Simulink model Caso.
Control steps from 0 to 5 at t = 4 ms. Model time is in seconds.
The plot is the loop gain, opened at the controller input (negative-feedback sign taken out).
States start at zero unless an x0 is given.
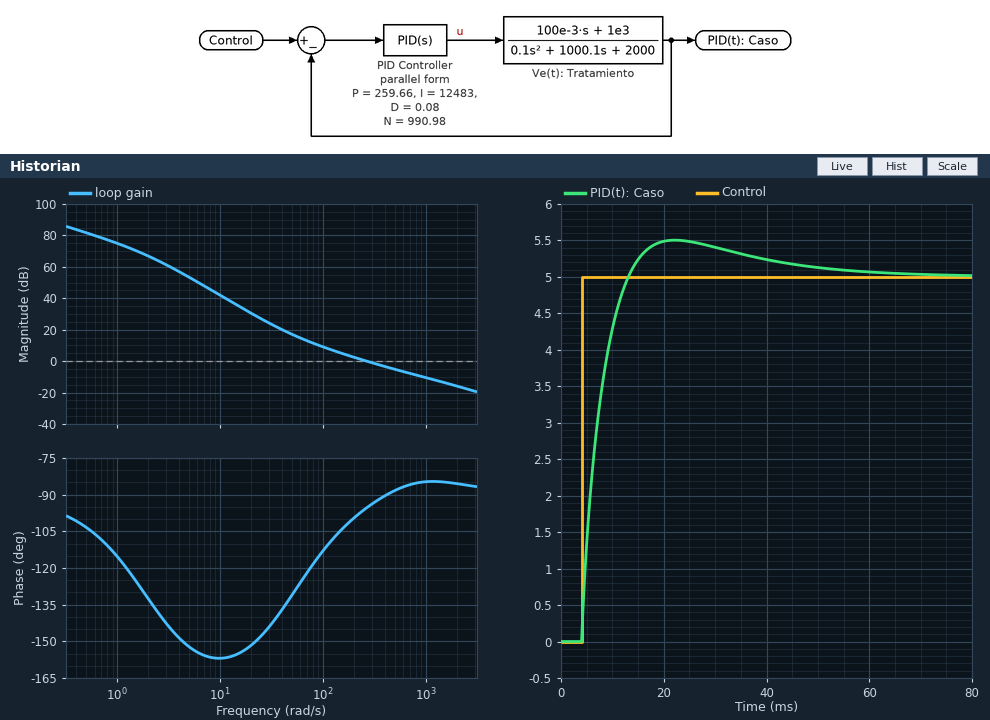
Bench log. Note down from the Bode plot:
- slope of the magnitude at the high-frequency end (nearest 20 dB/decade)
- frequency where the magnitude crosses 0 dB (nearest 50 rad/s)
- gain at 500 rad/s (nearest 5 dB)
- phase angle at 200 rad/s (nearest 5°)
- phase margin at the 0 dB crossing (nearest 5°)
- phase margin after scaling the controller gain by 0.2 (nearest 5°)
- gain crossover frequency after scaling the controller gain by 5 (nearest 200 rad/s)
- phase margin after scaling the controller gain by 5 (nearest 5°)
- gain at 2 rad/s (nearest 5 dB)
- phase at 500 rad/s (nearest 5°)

-20 dB/decade
250 rad/s
-5 dB
-100°
85°
55°
1600 rad/s
95°
65 dB
-90°
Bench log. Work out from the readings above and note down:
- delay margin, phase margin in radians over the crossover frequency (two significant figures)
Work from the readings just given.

0.0059 s
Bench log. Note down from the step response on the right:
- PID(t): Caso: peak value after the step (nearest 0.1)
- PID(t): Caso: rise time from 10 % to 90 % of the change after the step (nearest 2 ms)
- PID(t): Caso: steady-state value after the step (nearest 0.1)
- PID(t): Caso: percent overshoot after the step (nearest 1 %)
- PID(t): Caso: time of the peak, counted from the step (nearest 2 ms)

5.5
6 ms
5.0
10 %
18 ms
